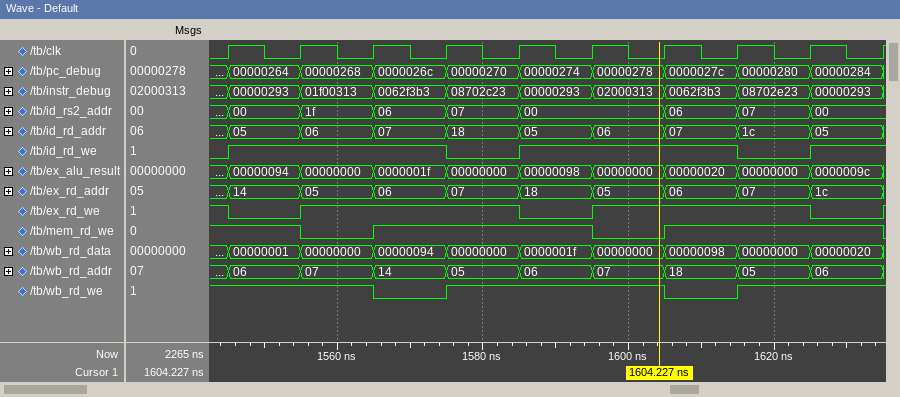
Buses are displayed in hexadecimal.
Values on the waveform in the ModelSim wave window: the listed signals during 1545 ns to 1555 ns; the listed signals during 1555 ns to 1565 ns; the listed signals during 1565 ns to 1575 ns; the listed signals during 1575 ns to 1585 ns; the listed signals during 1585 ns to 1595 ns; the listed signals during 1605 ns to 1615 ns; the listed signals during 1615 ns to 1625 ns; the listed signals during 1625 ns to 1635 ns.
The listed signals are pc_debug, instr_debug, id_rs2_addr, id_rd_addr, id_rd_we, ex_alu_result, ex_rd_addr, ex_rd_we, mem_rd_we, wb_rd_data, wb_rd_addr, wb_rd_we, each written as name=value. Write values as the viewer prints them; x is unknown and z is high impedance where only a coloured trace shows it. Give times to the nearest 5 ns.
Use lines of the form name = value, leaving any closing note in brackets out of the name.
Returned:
the listed signals during 1545 ns to 1555 ns = pc_debug=00000264, instr_debug=00000293, id_rs2_addr=00, id_rd_addr=05, id_rd_we=1, ex_alu_result=00000094, ex_rd_addr=14, ex_rd_we=0, mem_rd_we=1, wb_rd_data=00000001, wb_rd_addr=06, wb_rd_we=1
the listed signals during 1555 ns to 1565 ns = pc_debug=00000268, instr_debug=01f00313, id_rs2_addr=1f, id_rd_addr=06, id_rd_we=1, ex_alu_result=00000000, ex_rd_addr=05, ex_rd_we=1, mem_rd_we=0, wb_rd_data=00000000, wb_rd_addr=07, wb_rd_we=1
the listed signals during 1565 ns to 1575 ns = pc_debug=0000026c, instr_debug=0062f3b3, id_rs2_addr=06, id_rd_addr=07, id_rd_we=1, ex_alu_result=0000001f, ex_rd_addr=06, ex_rd_we=1, mem_rd_we=1, wb_rd_data=00000094, wb_rd_addr=14, wb_rd_we=0
the listed signals during 1575 ns to 1585 ns = pc_debug=00000270, instr_debug=08702c23, id_rs2_addr=07, id_rd_addr=18, id_rd_we=0, ex_alu_result=00000000, ex_rd_addr=07, ex_rd_we=1, mem_rd_we=1, wb_rd_data=00000000, wb_rd_addr=05, wb_rd_we=1
the listed signals during 1585 ns to 1595 ns = pc_debug=00000274, instr_debug=00000293, id_rs2_addr=00, id_rd_addr=05, id_rd_we=1, ex_alu_result=00000098, ex_rd_addr=18, ex_rd_we=0, mem_rd_we=1, wb_rd_data=0000001f, wb_rd_addr=06, wb_rd_we=1
the listed signals during 1605 ns to 1615 ns = pc_debug=0000027c, instr_debug=0062f3b3, id_rs2_addr=06, id_rd_addr=07, id_rd_we=1, ex_alu_result=00000020, ex_rd_addr=06, ex_rd_we=1, mem_rd_we=1, wb_rd_data=00000098, wb_rd_addr=18, wb_rd_we=0
the listed signals during 1615 ns to 1625 ns = pc_debug=00000280, instr_debug=08702e23, id_rs2_addr=07, id_rd_addr=1c, id_rd_we=0, ex_alu_result=00000000, ex_rd_addr=07, ex_rd_we=1, mem_rd_we=1, wb_rd_data=00000000, wb_rd_addr=05, wb_rd_we=1
the listed signals during 1625 ns to 1635 ns = pc_debug=00000284, instr_debug=00000293, id_rs2_addr=00, id_rd_addr=05, id_rd_we=1, ex_alu_result=0000009c, ex_rd_addr=1c, ex_rd_we=0, mem_rd_we=1, wb_rd_data=00000020, wb_rd_addr=06, wb_rd_we=1
